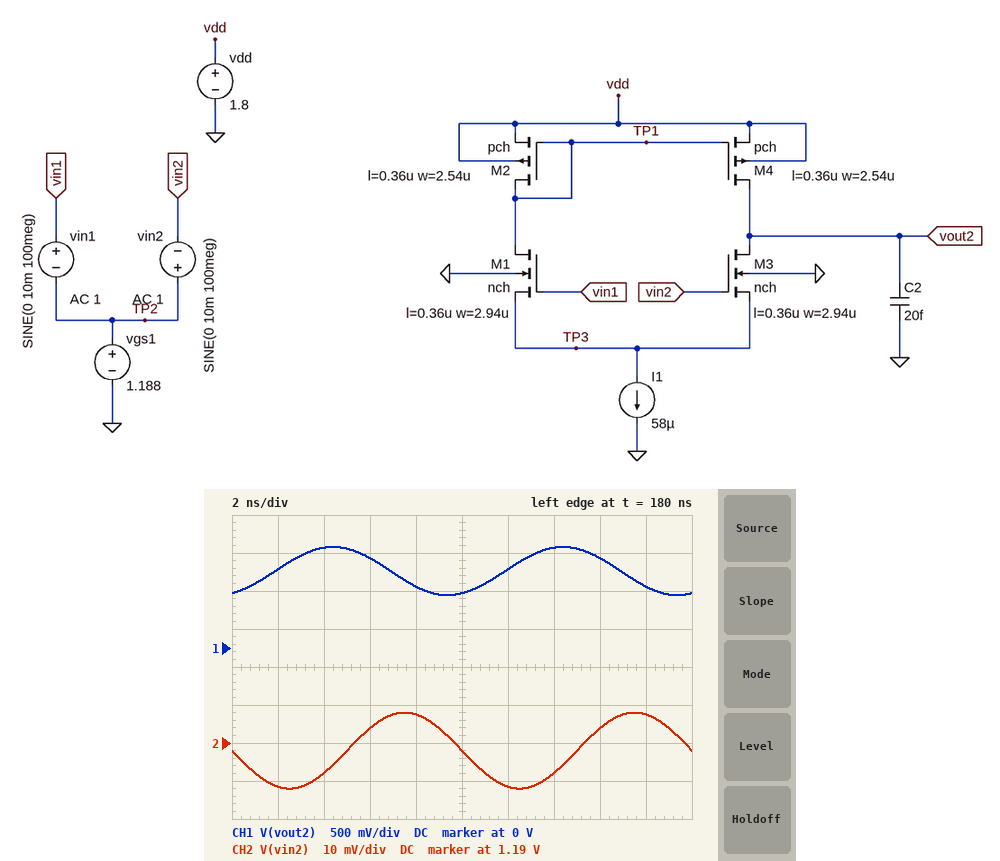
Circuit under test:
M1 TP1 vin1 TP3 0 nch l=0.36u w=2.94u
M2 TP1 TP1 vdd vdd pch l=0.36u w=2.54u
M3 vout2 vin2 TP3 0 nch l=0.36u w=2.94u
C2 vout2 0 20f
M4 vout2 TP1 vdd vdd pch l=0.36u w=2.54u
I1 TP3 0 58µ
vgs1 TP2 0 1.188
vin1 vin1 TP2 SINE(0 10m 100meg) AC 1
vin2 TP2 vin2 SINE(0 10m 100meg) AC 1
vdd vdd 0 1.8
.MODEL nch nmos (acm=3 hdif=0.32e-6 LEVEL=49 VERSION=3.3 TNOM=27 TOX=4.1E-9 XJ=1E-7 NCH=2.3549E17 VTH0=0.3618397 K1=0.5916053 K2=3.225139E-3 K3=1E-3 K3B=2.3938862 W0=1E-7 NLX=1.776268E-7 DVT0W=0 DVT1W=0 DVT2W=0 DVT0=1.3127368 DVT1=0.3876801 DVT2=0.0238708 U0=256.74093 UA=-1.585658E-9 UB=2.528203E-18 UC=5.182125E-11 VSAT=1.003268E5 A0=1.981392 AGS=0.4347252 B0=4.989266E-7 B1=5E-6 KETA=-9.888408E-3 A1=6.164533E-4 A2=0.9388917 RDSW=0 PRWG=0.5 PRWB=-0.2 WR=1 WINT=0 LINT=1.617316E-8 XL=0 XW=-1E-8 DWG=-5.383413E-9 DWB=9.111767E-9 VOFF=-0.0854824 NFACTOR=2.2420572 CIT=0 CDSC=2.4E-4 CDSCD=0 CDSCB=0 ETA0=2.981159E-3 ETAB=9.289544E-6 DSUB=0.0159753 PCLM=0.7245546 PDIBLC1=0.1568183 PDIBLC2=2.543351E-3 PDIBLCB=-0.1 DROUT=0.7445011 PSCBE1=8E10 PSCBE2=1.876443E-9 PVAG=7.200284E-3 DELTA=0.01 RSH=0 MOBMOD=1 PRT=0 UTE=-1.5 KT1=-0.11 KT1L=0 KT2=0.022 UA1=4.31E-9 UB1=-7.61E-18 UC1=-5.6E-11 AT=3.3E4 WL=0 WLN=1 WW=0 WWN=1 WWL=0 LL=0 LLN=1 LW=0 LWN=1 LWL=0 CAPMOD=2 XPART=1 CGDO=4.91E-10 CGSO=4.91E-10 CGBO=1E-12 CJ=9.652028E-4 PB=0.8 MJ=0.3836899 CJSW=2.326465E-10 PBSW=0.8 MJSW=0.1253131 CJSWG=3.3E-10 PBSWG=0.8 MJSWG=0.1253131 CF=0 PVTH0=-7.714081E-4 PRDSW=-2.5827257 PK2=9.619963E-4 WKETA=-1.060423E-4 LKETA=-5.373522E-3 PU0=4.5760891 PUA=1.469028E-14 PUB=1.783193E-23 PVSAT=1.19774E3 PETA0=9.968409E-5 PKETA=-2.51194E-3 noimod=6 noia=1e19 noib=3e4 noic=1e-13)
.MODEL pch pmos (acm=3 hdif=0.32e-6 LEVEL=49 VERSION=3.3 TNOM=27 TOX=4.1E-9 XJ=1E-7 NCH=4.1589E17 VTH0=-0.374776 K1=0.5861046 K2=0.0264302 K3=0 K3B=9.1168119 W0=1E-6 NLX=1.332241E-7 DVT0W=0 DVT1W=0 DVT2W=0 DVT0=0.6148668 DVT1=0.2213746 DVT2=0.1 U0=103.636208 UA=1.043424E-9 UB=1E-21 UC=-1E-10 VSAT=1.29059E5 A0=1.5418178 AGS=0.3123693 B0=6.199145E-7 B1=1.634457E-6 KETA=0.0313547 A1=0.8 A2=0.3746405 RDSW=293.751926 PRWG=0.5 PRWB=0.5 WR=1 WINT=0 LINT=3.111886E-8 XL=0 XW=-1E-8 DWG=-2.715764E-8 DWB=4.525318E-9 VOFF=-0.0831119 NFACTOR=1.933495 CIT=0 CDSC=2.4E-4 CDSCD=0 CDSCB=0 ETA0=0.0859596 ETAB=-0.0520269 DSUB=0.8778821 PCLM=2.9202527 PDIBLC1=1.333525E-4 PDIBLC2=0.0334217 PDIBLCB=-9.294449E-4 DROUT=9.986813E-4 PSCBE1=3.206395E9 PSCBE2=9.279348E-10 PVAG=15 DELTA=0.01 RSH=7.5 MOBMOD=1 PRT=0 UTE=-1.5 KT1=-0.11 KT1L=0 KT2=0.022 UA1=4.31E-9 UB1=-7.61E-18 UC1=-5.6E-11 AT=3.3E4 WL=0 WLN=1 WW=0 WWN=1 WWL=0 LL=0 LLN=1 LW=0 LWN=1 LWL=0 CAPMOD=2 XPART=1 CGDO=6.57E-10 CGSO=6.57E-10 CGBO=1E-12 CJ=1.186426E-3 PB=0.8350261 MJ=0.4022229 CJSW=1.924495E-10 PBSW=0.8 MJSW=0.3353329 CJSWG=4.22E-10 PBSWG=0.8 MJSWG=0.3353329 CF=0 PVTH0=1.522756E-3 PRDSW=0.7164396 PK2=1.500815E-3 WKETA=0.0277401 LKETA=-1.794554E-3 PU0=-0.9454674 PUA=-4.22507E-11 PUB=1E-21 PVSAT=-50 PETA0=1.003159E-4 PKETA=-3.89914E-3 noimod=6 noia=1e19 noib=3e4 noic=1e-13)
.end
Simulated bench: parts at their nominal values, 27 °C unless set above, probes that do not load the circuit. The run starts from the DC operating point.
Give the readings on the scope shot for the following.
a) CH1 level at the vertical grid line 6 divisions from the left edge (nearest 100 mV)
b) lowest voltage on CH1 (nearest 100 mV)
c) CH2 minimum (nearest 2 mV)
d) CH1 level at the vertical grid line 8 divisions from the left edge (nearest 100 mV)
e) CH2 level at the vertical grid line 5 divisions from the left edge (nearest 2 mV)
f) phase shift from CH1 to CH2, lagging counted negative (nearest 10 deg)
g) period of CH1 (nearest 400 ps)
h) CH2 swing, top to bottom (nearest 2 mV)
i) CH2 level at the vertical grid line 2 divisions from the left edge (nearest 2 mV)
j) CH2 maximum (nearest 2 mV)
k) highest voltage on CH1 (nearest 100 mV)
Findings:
1.0 V
700 mV
1.178 V
1.2 V
1.188 V
-110 deg
10.0 ns
20 mV
1.182 V
1.198 V
1.3 V
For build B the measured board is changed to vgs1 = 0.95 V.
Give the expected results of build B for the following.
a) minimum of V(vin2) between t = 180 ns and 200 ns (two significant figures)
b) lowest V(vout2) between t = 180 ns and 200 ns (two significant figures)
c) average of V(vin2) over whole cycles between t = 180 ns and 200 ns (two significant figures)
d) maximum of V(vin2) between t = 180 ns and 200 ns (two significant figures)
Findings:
940 mV
680 mV
950 mV
960 mV
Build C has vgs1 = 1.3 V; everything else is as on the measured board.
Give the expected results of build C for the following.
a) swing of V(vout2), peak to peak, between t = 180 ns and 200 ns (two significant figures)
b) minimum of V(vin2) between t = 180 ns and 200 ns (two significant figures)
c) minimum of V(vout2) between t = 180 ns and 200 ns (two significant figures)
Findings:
620 mV
1.3 V
720 mV
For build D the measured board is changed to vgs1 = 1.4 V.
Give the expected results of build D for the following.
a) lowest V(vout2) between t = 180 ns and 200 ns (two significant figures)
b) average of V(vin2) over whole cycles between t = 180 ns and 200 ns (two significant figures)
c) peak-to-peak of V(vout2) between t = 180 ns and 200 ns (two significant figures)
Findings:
760 mV
1.4 V
590 mV
